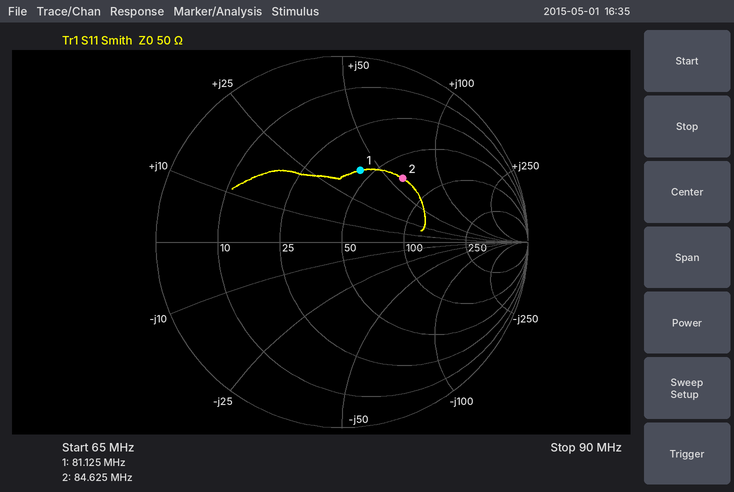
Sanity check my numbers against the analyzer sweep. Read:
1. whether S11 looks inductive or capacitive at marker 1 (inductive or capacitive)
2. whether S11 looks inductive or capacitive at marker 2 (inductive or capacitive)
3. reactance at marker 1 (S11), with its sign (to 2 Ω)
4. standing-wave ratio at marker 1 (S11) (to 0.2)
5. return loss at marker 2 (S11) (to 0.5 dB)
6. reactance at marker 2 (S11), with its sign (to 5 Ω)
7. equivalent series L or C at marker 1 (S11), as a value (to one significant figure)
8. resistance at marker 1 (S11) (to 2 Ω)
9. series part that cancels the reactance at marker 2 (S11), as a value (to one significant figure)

inductive
inductive
+40 Ω
2.4
6.5 dB
+60 Ω
80 nH
44 Ω
30 pF
